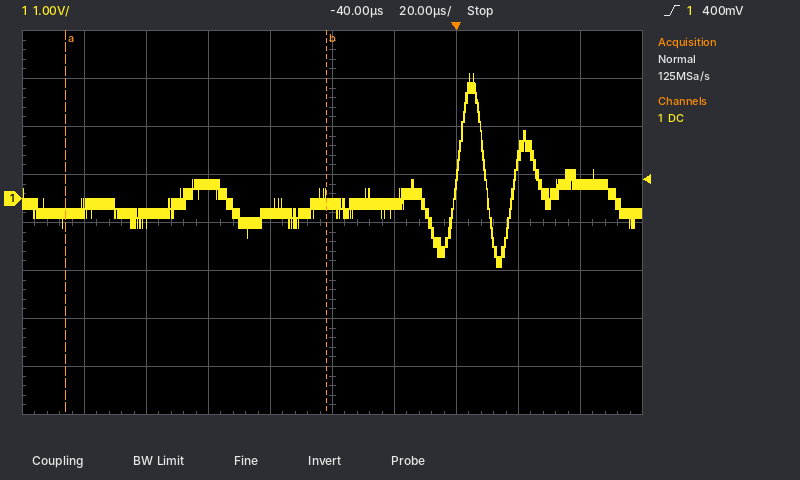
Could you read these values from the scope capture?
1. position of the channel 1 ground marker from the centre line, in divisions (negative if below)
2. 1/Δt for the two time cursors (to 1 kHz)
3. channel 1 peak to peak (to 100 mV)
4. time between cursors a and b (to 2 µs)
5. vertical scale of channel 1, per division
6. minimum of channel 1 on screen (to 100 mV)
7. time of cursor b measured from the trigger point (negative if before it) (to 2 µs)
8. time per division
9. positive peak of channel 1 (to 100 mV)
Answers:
+0.5 div
12 kHz
4.0 V
84 µs
1 V
-1.4 V
-42 µs
20 µs
2.6 V
